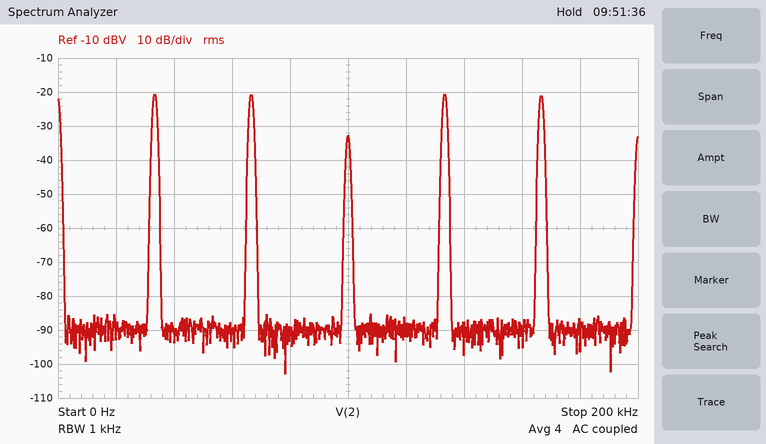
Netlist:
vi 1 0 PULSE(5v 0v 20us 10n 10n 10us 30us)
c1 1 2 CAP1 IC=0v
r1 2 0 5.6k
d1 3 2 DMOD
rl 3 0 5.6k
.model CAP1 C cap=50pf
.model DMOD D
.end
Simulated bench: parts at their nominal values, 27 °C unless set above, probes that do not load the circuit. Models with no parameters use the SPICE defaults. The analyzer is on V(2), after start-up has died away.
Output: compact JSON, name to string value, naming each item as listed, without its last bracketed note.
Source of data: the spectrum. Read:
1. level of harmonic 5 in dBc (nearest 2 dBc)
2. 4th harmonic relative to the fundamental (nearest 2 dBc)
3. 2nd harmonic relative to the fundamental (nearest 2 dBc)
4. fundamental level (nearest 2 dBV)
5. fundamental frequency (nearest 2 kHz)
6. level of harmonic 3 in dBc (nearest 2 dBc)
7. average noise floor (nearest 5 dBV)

{"level of harmonic 5 in dBc": "0 dBc", "4th harmonic relative to the fundamental": "0 dBc", "2nd harmonic relative to the fundamental": "0 dBc", "fundamental level": "-20 dBV", "fundamental frequency": "34 kHz", "level of harmonic 3 in dBc": "-12 dBc", "average noise floor": "-90 dBV"}
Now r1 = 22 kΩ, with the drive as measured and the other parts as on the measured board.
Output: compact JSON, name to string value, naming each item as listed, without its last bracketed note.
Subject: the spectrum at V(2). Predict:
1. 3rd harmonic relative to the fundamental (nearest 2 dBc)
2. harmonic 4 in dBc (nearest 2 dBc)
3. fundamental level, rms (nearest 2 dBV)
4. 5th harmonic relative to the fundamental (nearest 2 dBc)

{"3rd harmonic relative to the fundamental": "-8 dBc", "harmonic 4 in dBc": "-2 dBc", "fundamental level, rms": "-10 dBV", "5th harmonic relative to the fundamental": "-4 dBc"}
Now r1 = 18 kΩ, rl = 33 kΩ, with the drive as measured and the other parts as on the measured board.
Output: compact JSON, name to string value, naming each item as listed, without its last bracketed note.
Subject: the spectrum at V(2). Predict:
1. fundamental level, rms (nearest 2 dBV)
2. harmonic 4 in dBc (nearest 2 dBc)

{"fundamental level, rms": "-10 dBV", "harmonic 4 in dBc": "-2 dBc"}
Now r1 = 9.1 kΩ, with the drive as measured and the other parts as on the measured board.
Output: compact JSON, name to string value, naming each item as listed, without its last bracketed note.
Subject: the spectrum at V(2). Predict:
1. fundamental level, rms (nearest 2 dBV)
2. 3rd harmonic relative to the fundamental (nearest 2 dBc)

{"fundamental level, rms": "-16 dBV", "3rd harmonic relative to the fundamental": "-10 dBc"}
